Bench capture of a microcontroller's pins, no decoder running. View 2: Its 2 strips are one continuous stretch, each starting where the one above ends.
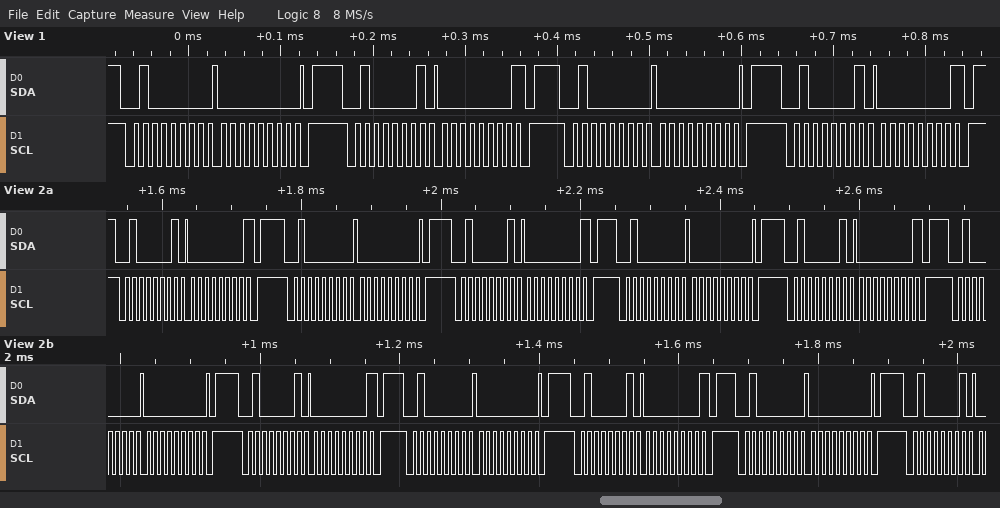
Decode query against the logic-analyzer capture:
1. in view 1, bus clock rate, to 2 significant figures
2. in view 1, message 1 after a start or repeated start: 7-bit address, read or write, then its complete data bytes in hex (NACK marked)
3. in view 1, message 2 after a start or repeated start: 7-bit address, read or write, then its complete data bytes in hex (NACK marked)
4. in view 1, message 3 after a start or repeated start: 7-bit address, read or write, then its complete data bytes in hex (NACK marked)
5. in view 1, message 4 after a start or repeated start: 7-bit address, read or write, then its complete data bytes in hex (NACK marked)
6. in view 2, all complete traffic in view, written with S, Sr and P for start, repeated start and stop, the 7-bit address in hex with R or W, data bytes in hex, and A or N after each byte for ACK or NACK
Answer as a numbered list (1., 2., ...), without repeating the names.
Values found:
1. 100 kHz
2. 0x20 write: 00
3. 0x20 read: 00 NACK
4. 0x20 write: 00
5. 0x20 read: 00 NACK
6. S 20R A 00 N P S 20W A 00 A P S 20R A 00 N P S 20W A 00 A P S 20R A 00 N P S 20W A 00 A P S 20R A 00 N P S 20W A 00 A P S 20R A 00 N P S 20W A 00 A P S 20R A
